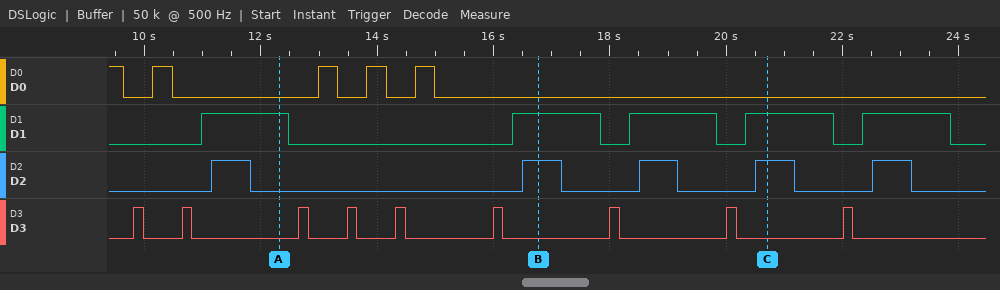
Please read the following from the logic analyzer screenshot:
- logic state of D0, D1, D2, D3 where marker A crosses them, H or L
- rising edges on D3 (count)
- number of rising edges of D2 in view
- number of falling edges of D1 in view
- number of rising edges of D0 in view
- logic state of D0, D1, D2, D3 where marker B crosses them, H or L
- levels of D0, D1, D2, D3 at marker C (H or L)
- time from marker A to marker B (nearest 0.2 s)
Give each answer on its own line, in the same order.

D0=L, D1=H, D2=L, D3=L
9
5
5
4
D0=L, D1=H, D2=H, D3=L
D0=L, D1=H, D2=H, D3=L
4.4 s
